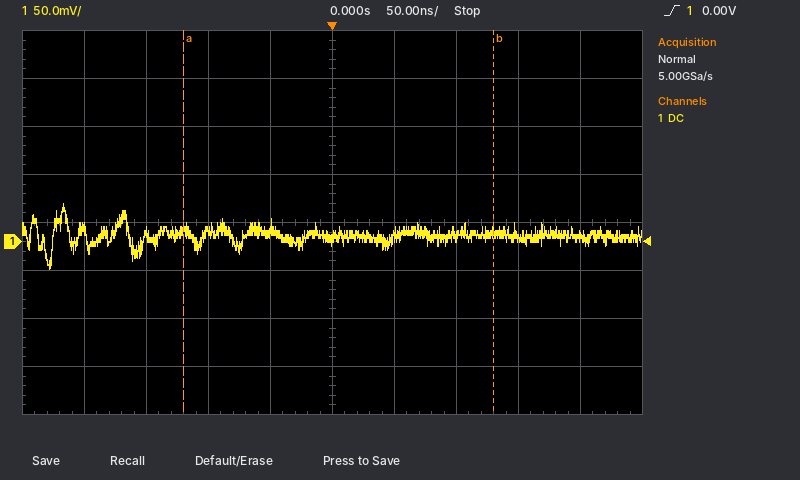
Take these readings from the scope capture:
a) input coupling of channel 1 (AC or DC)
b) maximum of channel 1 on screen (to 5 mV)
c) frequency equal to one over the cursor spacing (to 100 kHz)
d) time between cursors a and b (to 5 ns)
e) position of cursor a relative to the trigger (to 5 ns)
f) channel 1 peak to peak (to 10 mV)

DC
40 mV
4.0 MHz
250 ns
-120 ns
70 mV
